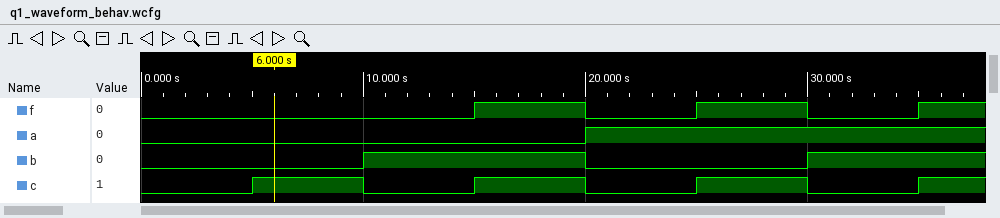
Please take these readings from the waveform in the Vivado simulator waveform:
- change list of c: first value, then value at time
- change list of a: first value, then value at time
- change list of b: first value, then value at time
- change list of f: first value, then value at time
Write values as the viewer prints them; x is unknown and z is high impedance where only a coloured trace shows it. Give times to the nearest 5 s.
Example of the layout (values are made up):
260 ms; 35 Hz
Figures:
0, 1 at 5 s, 0 at 10 s, 1 at 15 s, 0 at 20 s, 1 at 25 s, 0 at 30 s, 1 at 35 s; 0, 1 at 20 s; 0, 1 at 10 s, 0 at 20 s, 1 at 30 s; 0, 1 at 15 s, 0 at 20 s, 1 at 25 s, 0 at 30 s, 1 at 35 s
